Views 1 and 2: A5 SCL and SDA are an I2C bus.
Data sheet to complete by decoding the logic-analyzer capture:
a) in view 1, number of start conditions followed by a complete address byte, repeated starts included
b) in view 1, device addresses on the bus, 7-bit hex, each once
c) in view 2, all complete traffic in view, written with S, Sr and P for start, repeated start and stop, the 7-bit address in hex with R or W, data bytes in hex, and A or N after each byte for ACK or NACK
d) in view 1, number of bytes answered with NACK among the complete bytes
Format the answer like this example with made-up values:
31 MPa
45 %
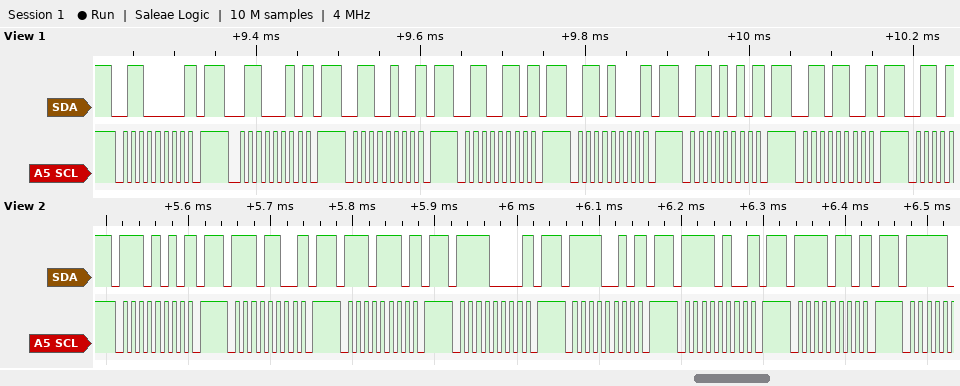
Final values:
7
0x30 0x31 0x32 0x33 0x34 0x35 0x36
S 75W N P S 76W N P S 77W N P S 78W N P S 79W N P S 7AW N P S 7BW N P
7
